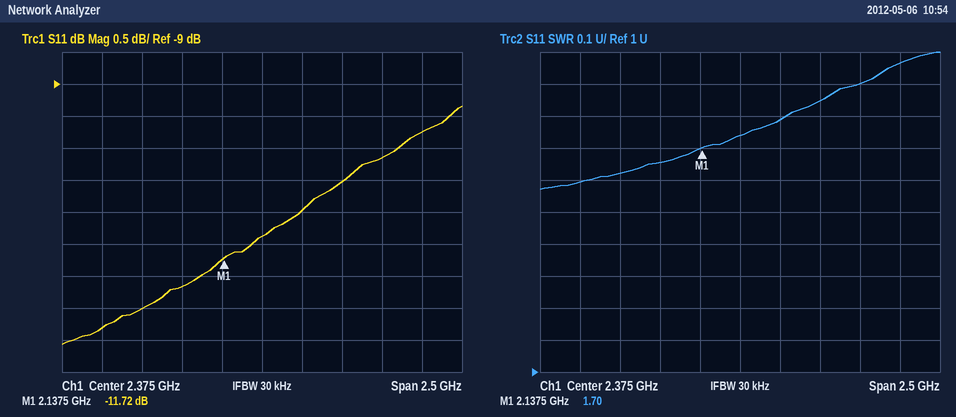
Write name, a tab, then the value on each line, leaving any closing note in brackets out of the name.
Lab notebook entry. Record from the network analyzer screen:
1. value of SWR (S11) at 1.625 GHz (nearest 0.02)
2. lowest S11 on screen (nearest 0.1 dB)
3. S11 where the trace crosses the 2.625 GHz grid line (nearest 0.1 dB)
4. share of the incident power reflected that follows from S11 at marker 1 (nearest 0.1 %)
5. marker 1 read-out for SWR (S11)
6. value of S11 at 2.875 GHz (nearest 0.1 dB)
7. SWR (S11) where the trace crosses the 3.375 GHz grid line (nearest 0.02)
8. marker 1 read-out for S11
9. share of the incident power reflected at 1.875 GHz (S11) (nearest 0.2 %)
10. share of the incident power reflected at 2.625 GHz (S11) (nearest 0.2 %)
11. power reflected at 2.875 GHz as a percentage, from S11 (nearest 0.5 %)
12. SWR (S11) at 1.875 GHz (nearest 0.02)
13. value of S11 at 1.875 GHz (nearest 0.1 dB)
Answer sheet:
value of SWR (S11) at 1.625 GHz	1.62
lowest S11 on screen	-13.1 dB
S11 where the trace crosses the 2.625 GHz grid line	-11.0 dB
share of the incident power reflected that follows from S11 at marker 1	6.7 %
marker 1 read-out for SWR	1.70
value of S11 at 2.875 GHz	-10.5 dB
SWR (S11) where the trace crosses the 3.375 GHz grid line	1.96
marker 1 read-out for S11	-11.72 dB
share of the incident power reflected at 1.875 GHz (S11)	6.0 %
share of the incident power reflected at 2.625 GHz (S11)	8.0 %
power reflected at 2.875 GHz as a percentage, from S11	9.0 %
SWR (S11) at 1.875 GHz	1.66
value of S11 at 1.875 GHz	-12.2 dB
